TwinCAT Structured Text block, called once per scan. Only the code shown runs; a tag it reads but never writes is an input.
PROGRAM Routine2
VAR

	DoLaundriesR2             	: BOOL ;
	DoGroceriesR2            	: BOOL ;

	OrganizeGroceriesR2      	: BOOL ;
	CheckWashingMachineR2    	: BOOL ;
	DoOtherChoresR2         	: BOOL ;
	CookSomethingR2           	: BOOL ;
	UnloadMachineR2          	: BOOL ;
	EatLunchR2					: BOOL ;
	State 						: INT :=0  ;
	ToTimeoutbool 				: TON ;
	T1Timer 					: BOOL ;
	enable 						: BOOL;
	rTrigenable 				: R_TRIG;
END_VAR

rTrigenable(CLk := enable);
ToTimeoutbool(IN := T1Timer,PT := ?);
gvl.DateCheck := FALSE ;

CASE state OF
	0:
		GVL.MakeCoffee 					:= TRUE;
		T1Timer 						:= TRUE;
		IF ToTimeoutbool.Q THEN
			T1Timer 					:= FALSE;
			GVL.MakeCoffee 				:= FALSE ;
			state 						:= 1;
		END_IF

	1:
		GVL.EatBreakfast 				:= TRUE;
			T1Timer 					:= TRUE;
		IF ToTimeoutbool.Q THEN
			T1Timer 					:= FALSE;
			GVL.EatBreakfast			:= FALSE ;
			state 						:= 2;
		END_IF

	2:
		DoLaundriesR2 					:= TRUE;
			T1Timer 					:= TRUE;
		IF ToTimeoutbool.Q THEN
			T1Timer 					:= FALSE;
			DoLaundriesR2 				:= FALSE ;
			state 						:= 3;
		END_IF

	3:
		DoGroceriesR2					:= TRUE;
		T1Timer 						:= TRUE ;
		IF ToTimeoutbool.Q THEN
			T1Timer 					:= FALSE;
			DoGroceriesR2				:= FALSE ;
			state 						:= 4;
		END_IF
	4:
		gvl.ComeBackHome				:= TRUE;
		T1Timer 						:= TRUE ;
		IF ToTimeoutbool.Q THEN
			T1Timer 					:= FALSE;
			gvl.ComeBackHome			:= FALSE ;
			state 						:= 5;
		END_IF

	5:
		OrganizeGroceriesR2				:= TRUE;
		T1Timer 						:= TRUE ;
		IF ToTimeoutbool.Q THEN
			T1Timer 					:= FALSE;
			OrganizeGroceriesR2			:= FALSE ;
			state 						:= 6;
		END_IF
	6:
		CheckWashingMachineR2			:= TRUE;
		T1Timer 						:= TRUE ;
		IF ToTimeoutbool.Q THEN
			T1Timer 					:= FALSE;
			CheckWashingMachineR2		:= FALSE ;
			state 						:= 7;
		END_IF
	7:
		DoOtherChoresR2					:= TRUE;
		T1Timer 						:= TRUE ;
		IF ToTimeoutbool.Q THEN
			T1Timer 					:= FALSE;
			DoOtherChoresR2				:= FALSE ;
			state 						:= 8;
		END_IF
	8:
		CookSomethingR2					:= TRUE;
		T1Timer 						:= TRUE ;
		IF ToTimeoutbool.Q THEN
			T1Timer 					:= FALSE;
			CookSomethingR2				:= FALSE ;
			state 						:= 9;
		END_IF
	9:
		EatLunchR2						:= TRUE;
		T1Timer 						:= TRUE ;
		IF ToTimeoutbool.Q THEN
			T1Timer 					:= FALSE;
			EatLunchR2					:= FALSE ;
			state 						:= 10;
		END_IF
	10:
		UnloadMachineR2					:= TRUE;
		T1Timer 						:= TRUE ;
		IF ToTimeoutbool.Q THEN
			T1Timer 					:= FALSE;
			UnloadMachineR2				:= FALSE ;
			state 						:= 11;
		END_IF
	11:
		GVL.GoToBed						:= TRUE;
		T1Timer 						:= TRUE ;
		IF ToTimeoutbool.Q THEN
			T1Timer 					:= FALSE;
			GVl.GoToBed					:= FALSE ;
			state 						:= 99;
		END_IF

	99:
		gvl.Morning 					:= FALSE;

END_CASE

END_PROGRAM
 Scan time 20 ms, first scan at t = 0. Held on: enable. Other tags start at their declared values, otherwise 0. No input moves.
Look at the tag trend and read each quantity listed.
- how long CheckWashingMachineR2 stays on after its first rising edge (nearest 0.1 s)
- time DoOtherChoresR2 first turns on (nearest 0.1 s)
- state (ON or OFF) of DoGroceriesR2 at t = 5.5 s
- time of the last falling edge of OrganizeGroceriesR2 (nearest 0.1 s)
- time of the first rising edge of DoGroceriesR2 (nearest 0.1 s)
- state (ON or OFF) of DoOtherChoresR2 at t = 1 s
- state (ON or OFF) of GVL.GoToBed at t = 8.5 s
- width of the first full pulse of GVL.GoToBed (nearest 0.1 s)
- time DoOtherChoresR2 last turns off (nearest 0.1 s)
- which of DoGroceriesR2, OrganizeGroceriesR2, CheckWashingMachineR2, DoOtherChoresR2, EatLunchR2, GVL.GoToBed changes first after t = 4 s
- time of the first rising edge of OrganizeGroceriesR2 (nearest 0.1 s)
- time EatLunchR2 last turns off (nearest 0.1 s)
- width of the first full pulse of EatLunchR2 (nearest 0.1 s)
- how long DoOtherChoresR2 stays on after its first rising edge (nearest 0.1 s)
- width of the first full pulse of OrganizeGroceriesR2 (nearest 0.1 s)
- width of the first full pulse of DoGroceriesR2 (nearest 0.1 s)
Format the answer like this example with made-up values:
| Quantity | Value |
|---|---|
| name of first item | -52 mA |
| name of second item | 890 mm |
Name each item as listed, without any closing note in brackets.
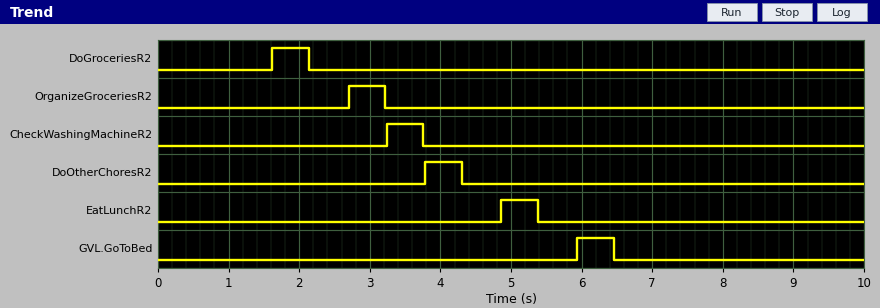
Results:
| Quantity | Value |
|---|---|
| how long CheckWashingMachineR2 stays on after its first rising edge | 0.5 s |
| time DoOtherChoresR2 first turns on | 3.8 s |
| state (ON or OFF) of DoGroceriesR2 at t = 5.5 s | OFF |
| time of the last falling edge of OrganizeGroceriesR2 | 3.2 s |
| time of the first rising edge of DoGroceriesR2 | 1.6 s |
| state (ON or OFF) of DoOtherChoresR2 at t = 1 s | OFF |
| state (ON or OFF) of GVL.GoToBed at t = 8.5 s | OFF |
| width of the first full pulse of GVL.GoToBed | 0.5 s |
| time DoOtherChoresR2 last turns off | 4.3 s |
| which of DoGroceriesR2, OrganizeGroceriesR2, CheckWashingMachineR2, DoOtherChoresR2, EatLunchR2, GVL.GoToBed changes first after t = 4 s | DoOtherChoresR2 |
| time of the first rising edge of OrganizeGroceriesR2 | 2.7 s |
| time EatLunchR2 last turns off | 5.4 s |
| width of the first full pulse of EatLunchR2 | 0.5 s |
| how long DoOtherChoresR2 stays on after its first rising edge | 0.5 s |
| width of the first full pulse of OrganizeGroceriesR2 | 0.5 s |
| width of the first full pulse of DoGroceriesR2 | 0.5 s |
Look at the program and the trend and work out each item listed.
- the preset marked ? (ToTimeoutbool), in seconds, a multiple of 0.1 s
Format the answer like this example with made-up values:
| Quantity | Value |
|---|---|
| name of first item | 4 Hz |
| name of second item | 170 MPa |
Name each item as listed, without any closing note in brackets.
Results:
| Quantity | Value |
|---|---|
| the preset marked ? (ToTimeoutbool), in seconds, a multiple of 0.1 s | 0.5 s |
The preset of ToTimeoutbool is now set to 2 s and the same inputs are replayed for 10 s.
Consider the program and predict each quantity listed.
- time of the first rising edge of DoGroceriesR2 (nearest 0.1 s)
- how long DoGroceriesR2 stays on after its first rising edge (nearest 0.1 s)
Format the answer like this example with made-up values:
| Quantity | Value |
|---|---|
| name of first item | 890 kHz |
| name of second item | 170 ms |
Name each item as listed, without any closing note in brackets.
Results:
| Quantity | Value |
|---|---|
| time of the first rising edge of DoGroceriesR2 | 6.1 s |
| how long DoGroceriesR2 stays on after its first rising edge | 2.0 s |
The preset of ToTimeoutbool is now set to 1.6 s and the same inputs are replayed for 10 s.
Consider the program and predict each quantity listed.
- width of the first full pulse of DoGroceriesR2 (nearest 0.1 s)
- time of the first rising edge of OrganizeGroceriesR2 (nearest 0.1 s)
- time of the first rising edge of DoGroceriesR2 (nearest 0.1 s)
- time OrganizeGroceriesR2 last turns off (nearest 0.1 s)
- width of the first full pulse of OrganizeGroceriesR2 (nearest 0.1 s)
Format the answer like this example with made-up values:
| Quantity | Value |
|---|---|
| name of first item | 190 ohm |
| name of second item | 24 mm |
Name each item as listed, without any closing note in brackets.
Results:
| Quantity | Value |
|---|---|
| width of the first full pulse of DoGroceriesR2 | 1.6 s |
| time of the first rising edge of OrganizeGroceriesR2 | 8.2 s |
| time of the first rising edge of DoGroceriesR2 | 4.9 s |
| time OrganizeGroceriesR2 last turns off | 9.8 s |
| width of the first full pulse of OrganizeGroceriesR2 | 1.6 s |
